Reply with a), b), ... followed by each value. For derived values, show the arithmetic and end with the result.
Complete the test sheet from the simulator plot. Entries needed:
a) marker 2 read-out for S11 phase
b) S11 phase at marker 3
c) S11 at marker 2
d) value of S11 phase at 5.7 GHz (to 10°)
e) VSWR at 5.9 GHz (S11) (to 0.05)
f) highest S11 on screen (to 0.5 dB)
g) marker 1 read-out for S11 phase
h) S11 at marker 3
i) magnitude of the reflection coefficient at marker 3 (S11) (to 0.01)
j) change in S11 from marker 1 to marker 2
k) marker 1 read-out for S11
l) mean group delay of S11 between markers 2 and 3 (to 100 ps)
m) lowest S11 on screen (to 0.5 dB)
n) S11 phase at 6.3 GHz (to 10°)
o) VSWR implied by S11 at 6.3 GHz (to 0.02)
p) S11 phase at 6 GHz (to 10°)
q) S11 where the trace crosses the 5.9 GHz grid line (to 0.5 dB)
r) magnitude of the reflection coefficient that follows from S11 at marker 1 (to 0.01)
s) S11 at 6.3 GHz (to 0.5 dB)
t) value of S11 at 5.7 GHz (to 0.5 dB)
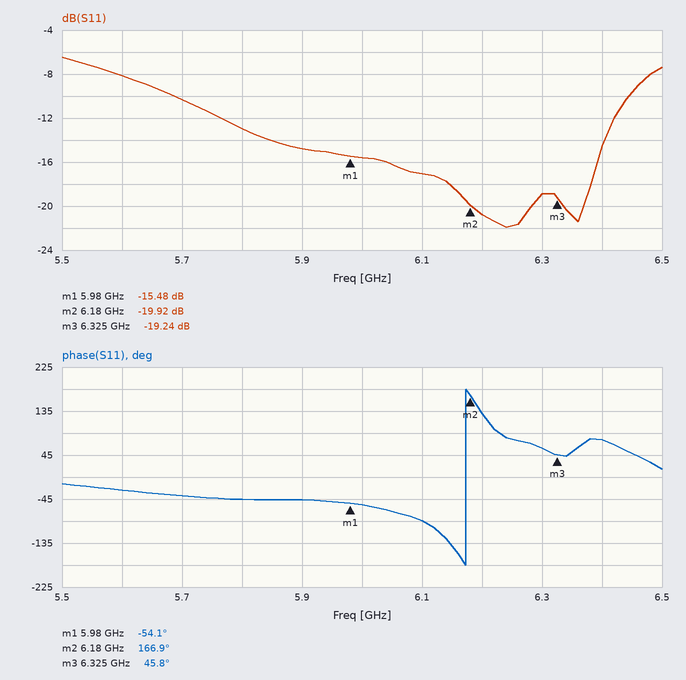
a) 166.9°
b) 45.8°
c) -19.92 dB
d) -40°
e) |Γ| = 10^(-15/20) = 0.1778; VSWR = (1 + 0.1778)/(1 − 0.1778) ≈ 1.43, so 1.45 to the nearest 0.05
f) -6.5 dB
g) -54.1°
h) -19.24 dB
i) 10^(-19.24/20) ≈ 0.11
j) -19.92 − (-15.48) = -4.44 dB
k) -15.48 dB
l) −(45.8° − (166.9°))/(360° × 145 MHz) ≈ 2.3 ns
m) -22.0 dB
n) 60°
o) |Γ| = 10^(-19/20) = 0.1122; VSWR = (1 + 0.1122)/(1 − 0.1122) ≈ 1.25, so 1.26 to the nearest 0.02
p) -60°
q) -15.0 dB
r) 10^(-15.48/20) ≈ 0.17
s) -19.0 dB
t) -10.5 dB
